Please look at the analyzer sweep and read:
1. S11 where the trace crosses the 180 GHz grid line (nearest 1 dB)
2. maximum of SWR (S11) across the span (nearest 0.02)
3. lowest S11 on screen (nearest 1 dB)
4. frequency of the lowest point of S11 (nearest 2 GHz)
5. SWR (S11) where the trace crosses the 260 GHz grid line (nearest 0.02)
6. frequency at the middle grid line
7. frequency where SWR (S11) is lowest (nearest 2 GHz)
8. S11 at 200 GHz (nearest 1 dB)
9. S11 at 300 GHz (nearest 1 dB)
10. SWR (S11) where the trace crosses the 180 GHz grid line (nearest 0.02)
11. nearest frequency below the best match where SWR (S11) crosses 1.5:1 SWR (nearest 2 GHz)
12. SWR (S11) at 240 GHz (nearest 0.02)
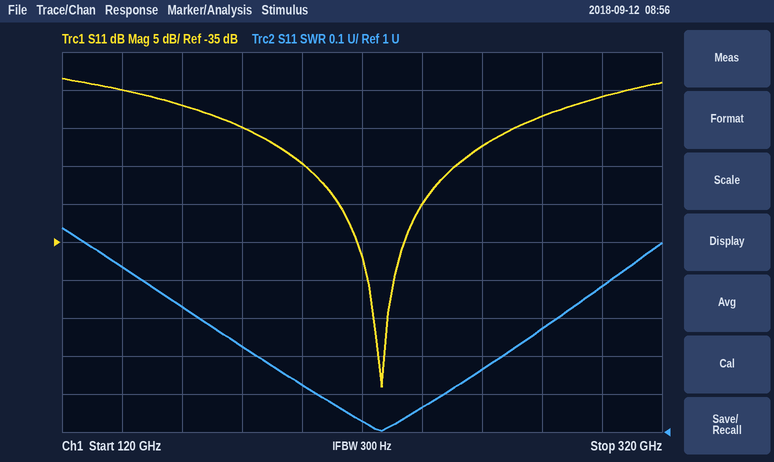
-20 dB
1.54
-54 dB
226 GHz
1.16
220 GHz
226 GHz
-25 dB
-16 dB
1.22
128 GHz
1.06
